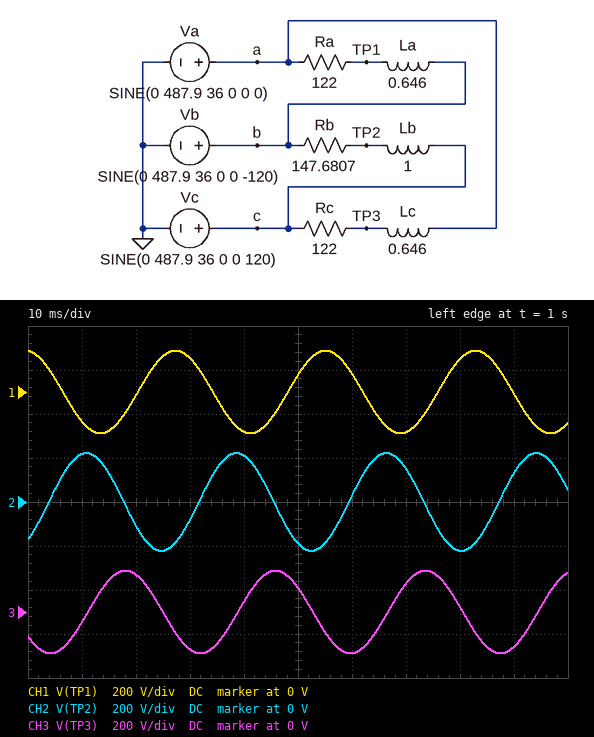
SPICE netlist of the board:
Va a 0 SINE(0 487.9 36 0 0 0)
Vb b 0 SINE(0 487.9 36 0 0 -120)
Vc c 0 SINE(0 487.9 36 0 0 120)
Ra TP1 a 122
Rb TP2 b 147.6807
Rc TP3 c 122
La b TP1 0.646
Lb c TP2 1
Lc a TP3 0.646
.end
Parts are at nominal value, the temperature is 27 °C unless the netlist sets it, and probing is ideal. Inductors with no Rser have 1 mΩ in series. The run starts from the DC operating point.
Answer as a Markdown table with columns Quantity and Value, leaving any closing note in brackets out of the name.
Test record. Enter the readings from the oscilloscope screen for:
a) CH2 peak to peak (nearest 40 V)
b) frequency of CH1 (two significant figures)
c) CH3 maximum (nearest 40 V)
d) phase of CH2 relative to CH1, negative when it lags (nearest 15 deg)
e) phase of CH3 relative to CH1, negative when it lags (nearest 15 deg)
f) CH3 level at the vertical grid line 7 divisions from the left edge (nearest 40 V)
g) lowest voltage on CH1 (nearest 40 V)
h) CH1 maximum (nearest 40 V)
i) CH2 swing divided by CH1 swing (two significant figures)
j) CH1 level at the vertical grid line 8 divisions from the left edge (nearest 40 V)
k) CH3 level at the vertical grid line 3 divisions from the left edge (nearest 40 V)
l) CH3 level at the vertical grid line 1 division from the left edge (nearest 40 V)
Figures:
| Quantity | Value |
|---|---|
| CH2 peak to peak | 440 V |
| frequency of CH1 | 36 Hz |
| CH3 maximum | 200 V |
| phase of CH2 relative to CH1, negative when it lags | -150 deg |
| phase of CH3 relative to CH1, negative when it lags | 120 deg |
| CH3 level at the vertical grid line 7 divisions from the left edge | 120 V |
| lowest voltage on CH1 | -200 V |
| CH1 maximum | 200 V |
| CH2 swing divided by CH1 swing | 1.2 |
| CH1 level at the vertical grid line 8 divisions from the left edge | 160 V |
| CH3 level at the vertical grid line 3 divisions from the left edge | -160 V |
| CH3 level at the vertical grid line 1 division from the left edge | -40 V |
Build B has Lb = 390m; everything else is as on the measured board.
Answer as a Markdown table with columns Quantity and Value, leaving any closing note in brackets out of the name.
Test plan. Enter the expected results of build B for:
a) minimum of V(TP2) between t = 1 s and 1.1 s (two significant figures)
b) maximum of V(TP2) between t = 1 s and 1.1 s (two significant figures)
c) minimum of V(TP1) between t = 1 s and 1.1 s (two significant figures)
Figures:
| Quantity | Value |
|---|---|
| minimum of V(TP2) between t = 1 s and 1.1 s | -240 V |
| maximum of V(TP2) between t = 1 s and 1.1 s | 240 V |
| minimum of V(TP1) between t = 1 s and 1.1 s | -190 V |
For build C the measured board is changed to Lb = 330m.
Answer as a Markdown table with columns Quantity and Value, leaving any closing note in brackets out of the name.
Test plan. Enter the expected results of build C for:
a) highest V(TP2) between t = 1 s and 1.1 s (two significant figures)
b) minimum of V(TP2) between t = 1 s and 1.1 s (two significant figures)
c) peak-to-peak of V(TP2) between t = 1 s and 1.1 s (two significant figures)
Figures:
| Quantity | Value |
|---|---|
| highest V(TP2) between t = 1 s and 1.1 s | 270 V |
| minimum of V(TP2) between t = 1 s and 1.1 s | -270 V |
| peak-to-peak of V(TP2) between t = 1 s and 1.1 s | 540 V |
